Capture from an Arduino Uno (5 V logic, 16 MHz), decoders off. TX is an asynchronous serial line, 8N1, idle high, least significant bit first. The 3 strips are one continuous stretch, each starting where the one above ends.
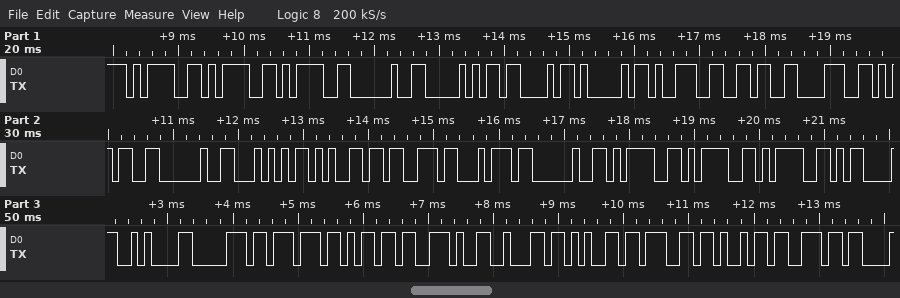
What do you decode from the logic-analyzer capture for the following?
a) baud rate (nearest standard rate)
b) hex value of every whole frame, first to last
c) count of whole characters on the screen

9600 baud
0x3D 0x3D 0x3D 0x20 0x50 0x43 0x41 0x39 0x36 0x38 0x35 0x20 0x54 0x65 0x73 0x74 0x20 0x3D 0x3D 0x3D 0x0D 0x0A 0x70 0x77 0x6D 0x2E 0x62 0x65 0x67 0x69 0x6E
31
